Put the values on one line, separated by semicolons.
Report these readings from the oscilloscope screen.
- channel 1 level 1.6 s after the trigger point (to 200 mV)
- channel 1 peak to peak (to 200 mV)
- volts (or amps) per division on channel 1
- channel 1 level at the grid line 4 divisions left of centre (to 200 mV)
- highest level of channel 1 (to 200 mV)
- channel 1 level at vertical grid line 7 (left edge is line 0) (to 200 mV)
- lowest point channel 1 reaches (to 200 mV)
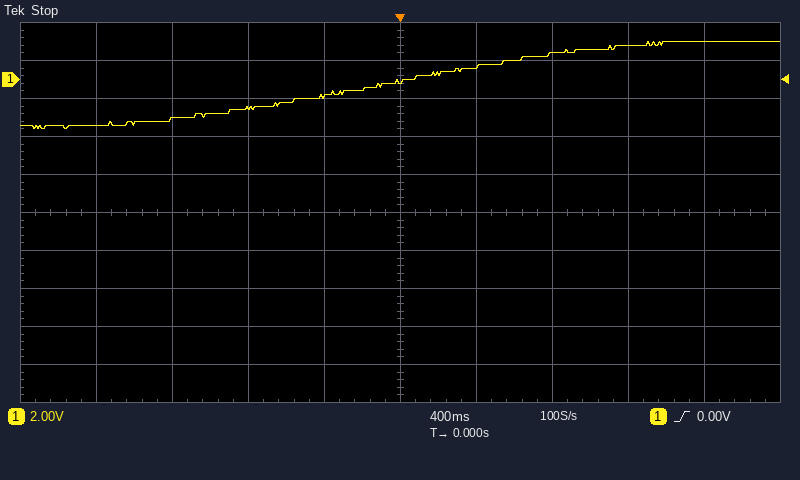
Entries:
2.0 V; 4.6 V; 2 V; -2.4 V; 2.0 V; 1.4 V; -2.6 V
